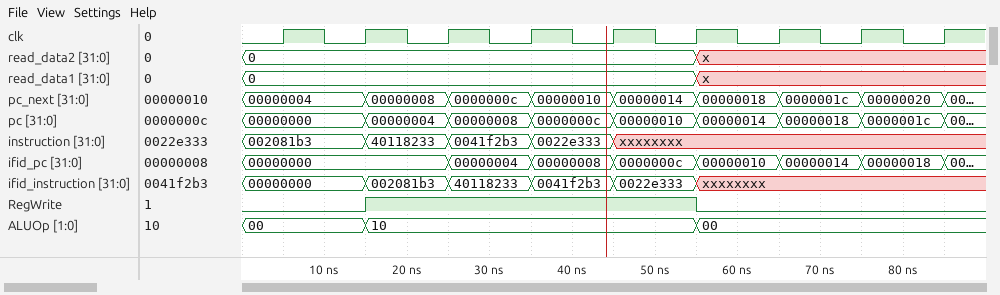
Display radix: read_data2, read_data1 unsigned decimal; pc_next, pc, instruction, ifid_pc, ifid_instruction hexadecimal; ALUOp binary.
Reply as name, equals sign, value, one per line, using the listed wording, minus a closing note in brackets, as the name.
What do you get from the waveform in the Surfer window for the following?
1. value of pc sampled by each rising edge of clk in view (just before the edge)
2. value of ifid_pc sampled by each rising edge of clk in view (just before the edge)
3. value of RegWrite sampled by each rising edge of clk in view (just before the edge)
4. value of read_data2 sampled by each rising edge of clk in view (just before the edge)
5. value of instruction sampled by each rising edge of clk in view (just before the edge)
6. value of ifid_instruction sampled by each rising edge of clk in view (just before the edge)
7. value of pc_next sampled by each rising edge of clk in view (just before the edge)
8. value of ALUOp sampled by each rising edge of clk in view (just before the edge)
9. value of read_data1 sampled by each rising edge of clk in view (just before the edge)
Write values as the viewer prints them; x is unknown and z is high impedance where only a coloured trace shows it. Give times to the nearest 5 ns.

value of pc sampled by each rising edge of clk in view = 00000000, 00000000, 00000004, 00000008, 0000000c, 00000010, 00000014, 00000018, 0000001c
value of ifid_pc sampled by each rising edge of clk in view = 00000000, 00000000, 00000000, 00000004, 00000008, 0000000c, 00000010, 00000014, 00000018
value of RegWrite sampled by each rising edge of clk in view = 0 0 1 1 1 1 0 0 0
value of read_data2 sampled by each rising edge of clk in view = 0, 0, 0, 0, 0, 0, x, x, x
value of instruction sampled by each rising edge of clk in view = 002081b3, 002081b3, 40118233, 0041f2b3, 0022e333, xxxxxxxx, xxxxxxxx, xxxxxxxx, xxxxxxxx
value of ifid_instruction sampled by each rising edge of clk in view = 00000000, 00000000, 002081b3, 40118233, 0041f2b3, 0022e333, xxxxxxxx, xxxxxxxx, xxxxxxxx
value of pc_next sampled by each rising edge of clk in view = 00000004, 00000004, 00000008, 0000000c, 00000010, 00000014, 00000018, 0000001c, 00000020
value of ALUOp sampled by each rising edge of clk in view = 00, 00, 10, 10, 10, 10, 00, 00, 00
value of read_data1 sampled by each rising edge of clk in view = 0, 0, 0, 0, 0, 0, x, x, x
